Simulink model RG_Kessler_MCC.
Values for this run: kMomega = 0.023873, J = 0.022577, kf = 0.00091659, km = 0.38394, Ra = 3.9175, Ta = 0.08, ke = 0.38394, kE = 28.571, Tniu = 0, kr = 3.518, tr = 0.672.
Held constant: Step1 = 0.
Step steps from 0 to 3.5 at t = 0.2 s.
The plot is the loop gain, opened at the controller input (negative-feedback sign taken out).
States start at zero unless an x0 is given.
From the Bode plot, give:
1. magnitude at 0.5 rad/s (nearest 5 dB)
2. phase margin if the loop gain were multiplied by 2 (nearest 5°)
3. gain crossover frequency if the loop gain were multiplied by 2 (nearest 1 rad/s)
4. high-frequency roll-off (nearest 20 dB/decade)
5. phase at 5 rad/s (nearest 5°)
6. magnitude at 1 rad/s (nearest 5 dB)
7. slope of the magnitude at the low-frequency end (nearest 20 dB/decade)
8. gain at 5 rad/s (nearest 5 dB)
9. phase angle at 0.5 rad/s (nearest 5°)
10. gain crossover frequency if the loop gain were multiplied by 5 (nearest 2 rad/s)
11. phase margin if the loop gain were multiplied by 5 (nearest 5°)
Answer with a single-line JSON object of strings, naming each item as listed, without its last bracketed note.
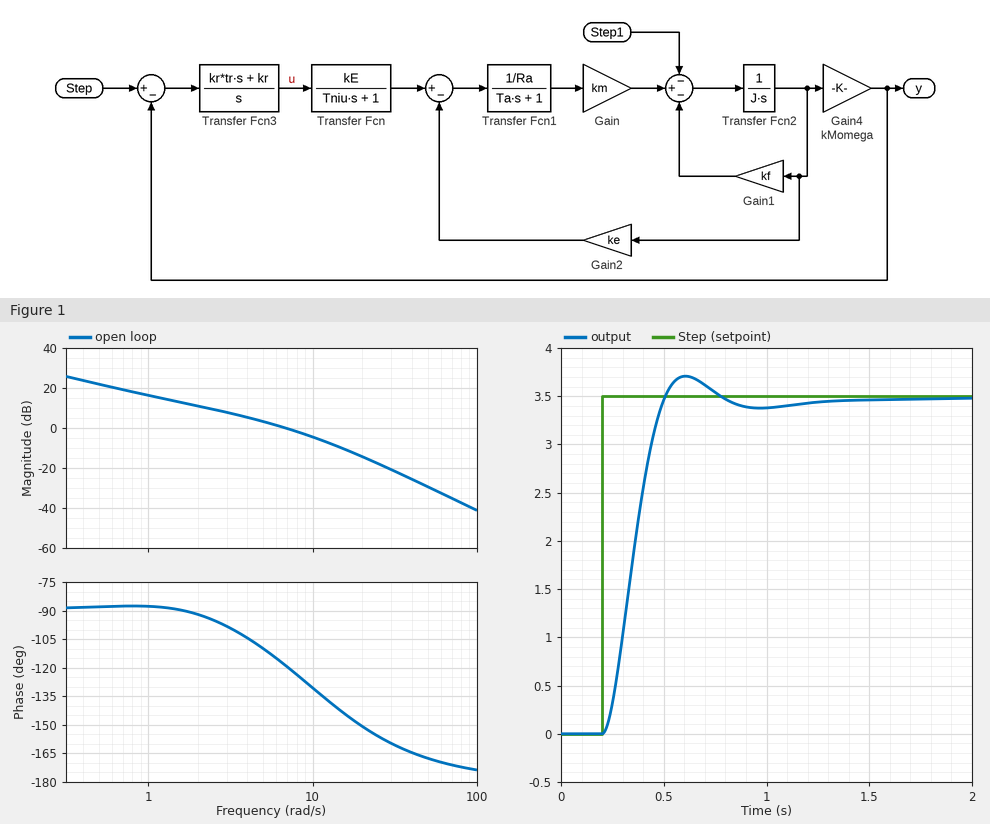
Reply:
{"magnitude at 0.5 rad/s": "20 dB", "phase margin if the loop gain were multiplied by 2": "45°", "gain crossover frequency if the loop gain were multiplied by 2": "11 rad/s", "high-frequency roll-off": "-40 dB/decade", "phase at 5 rad/s": "-110°", "magnitude at 1 rad/s": "15 dB", "slope of the magnitude at the low-frequency end": "-20 dB/decade", "gain at 5 rad/s": "5 dB", "phase angle at 0.5 rad/s": "-90°", "gain crossover frequency if the loop gain were multiplied by 5": "20 rad/s", "phase margin if the loop gain were multiplied by 5": "30°"}
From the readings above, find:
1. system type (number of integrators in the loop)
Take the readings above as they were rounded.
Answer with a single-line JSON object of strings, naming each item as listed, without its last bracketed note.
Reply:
{"system type": "1"}
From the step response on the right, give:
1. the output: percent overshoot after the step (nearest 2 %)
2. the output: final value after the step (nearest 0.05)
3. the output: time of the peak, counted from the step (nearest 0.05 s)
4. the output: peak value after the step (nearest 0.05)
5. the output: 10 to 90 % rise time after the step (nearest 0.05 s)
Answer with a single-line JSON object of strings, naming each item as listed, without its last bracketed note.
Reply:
{"the output: percent overshoot after the step": "6 %", "the output: final value after the step": "3.50", "the output: time of the peak, counted from the step": "0.40 s", "the output: peak value after the step": "3.70", "the output: 10 to 90 % rise time after the step": "0.20 s"}
